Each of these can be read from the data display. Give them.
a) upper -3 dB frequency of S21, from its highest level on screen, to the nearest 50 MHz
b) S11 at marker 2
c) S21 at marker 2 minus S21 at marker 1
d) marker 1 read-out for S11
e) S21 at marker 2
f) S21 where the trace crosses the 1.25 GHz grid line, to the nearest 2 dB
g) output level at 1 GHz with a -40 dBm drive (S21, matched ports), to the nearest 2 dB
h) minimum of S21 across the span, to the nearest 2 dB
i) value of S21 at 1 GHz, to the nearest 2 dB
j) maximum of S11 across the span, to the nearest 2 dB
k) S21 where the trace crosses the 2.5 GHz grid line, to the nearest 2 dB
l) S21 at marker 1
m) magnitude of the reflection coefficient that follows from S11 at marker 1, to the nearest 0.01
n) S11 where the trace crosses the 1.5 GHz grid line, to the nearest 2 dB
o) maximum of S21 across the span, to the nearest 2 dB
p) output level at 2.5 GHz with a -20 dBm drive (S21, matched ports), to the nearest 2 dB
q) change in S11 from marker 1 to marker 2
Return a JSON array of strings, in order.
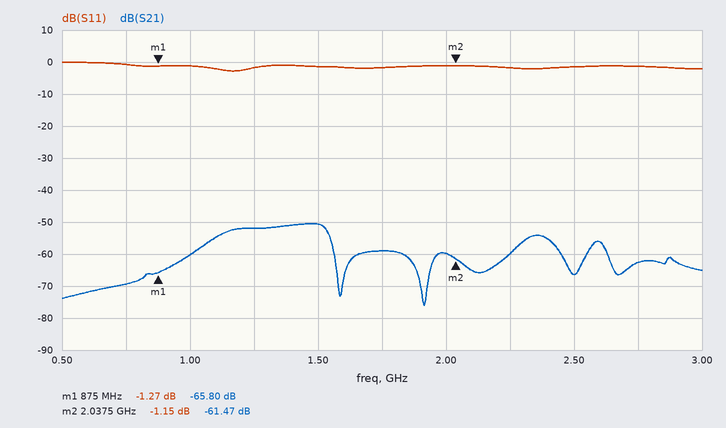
["1.55 GHz", "-1.15 dB", "4.33 dB", "-1.27 dB", "-61.47 dB", "-52 dB", "-100 dBm", "-76 dB", "-60 dB", "0 dB", "-66 dB", "-65.80 dB", "0.86", "-2 dB", "-50 dB", "-86 dBm", "0.12 dB"]
